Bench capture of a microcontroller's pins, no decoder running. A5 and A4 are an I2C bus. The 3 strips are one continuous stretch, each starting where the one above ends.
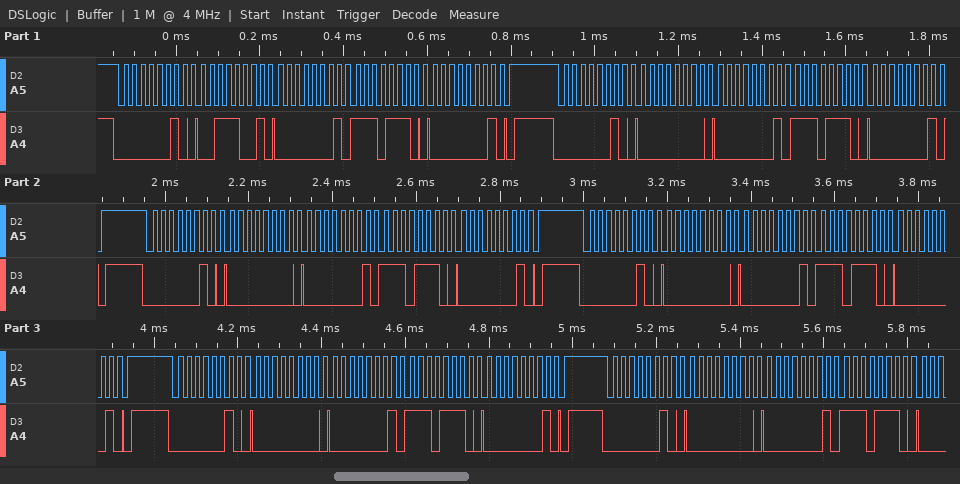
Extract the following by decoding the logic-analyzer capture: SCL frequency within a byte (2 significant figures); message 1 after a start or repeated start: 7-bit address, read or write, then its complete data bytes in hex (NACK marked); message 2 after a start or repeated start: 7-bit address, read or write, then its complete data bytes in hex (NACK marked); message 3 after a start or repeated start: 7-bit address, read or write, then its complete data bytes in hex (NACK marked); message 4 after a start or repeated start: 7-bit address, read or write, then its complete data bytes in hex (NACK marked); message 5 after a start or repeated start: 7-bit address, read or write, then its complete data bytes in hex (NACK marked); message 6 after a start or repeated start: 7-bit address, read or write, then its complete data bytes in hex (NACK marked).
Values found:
50 kHz
0x01 write: 39 01 EE 01
0x01 write: 00 01 EE 01
0x01 write: 00 01 EE 01
0x01 write: 00 01 EE 01
0x01 write: 00 01 EE 01
0x01 write: 00 01 EE
